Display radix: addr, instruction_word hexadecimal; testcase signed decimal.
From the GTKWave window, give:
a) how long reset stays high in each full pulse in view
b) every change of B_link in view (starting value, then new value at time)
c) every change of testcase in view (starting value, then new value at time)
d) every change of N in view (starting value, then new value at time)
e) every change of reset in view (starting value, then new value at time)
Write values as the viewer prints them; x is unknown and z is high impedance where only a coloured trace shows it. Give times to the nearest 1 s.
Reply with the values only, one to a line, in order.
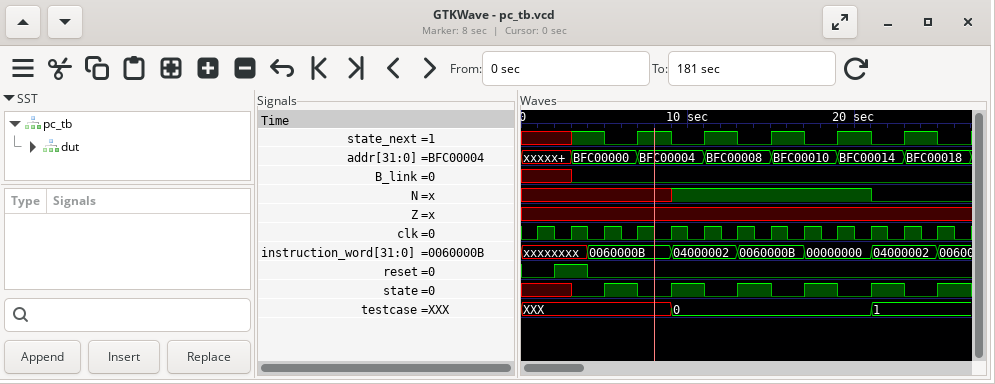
2 s
x, 0 at 3 s
XXX, 0 at 9 s, 1 at 21 s
x, 1 at 9 s, 0 at 21 s
0, 1 at 2 s, 0 at 4 s
